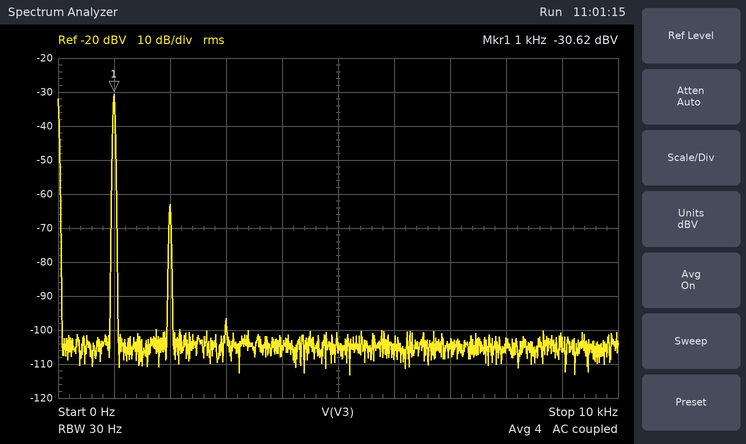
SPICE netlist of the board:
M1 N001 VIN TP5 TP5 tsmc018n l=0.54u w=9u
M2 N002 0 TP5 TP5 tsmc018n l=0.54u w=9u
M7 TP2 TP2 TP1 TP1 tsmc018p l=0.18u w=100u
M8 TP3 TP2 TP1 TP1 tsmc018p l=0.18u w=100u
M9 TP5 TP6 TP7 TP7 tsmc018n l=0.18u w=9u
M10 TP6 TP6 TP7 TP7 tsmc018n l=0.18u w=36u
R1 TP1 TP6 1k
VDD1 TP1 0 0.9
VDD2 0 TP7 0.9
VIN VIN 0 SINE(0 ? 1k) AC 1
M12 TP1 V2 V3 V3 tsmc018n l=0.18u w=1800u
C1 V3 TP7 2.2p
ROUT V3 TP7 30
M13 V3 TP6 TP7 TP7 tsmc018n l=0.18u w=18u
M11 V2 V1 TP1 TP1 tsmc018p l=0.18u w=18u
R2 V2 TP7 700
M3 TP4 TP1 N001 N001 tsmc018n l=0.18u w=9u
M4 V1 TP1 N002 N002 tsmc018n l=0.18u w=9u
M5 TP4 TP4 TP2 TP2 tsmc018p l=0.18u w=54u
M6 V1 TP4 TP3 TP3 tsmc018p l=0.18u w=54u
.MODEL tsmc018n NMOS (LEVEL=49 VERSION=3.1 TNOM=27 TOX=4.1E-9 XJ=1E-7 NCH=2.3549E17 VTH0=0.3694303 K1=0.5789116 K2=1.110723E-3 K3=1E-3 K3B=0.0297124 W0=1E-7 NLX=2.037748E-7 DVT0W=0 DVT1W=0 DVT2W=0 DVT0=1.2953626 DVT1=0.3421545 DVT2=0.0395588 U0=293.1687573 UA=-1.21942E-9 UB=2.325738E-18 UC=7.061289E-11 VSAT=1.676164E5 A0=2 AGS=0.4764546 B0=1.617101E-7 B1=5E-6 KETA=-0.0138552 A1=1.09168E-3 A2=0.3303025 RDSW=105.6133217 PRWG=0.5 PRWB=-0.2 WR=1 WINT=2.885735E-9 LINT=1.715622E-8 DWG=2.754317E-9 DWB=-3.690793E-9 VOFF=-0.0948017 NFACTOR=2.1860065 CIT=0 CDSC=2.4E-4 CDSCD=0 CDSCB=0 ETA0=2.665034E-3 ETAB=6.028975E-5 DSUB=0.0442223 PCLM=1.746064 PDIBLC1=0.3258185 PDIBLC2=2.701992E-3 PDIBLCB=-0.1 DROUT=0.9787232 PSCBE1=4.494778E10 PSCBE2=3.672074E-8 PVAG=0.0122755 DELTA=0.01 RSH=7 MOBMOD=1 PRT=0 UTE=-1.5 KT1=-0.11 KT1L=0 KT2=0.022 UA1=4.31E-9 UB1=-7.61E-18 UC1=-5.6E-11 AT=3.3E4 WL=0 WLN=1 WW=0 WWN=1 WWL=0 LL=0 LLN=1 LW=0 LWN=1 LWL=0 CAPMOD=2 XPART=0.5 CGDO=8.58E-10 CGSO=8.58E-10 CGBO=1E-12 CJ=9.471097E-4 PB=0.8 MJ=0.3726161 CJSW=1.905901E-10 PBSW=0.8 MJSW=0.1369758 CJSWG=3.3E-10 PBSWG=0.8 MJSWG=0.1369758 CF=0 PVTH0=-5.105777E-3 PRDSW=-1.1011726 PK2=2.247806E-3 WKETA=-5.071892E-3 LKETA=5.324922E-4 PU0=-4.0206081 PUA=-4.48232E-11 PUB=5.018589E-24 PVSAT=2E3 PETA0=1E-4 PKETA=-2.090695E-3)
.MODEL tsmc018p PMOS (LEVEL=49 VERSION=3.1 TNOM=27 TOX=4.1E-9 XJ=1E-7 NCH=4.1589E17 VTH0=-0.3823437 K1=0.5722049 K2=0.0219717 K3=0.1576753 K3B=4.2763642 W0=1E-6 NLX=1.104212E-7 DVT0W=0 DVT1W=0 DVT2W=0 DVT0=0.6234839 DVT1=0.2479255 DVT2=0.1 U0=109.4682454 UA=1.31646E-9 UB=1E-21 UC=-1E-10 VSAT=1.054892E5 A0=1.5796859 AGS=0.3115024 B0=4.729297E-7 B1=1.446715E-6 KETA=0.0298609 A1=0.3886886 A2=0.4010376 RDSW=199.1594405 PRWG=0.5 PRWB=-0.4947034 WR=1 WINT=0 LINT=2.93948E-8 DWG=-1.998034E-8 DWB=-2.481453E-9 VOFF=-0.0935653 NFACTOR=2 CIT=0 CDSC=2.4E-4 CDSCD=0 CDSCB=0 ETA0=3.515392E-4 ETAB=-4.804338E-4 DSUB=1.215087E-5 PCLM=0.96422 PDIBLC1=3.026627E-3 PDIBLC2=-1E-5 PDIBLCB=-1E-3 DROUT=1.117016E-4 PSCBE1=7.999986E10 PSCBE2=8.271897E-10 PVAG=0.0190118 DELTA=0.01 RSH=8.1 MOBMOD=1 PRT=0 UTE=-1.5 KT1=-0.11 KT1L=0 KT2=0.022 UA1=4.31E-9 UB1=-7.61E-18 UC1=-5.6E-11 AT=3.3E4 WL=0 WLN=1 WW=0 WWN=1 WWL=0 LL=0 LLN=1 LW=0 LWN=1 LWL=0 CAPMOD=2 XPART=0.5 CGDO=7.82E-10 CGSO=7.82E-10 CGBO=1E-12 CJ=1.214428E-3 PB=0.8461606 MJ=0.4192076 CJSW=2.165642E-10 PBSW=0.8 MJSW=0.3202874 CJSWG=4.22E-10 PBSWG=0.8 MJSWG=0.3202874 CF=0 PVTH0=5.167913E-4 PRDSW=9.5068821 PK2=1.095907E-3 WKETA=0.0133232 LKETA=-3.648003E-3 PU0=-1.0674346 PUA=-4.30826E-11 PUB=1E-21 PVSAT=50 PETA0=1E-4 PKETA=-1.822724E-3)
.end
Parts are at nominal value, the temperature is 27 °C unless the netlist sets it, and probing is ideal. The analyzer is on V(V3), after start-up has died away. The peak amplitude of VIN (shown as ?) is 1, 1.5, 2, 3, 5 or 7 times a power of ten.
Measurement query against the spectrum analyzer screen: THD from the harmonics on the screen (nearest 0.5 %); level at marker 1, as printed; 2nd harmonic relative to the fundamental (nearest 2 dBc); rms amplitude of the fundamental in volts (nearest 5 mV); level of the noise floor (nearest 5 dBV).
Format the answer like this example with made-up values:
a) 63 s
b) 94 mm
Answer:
a) 2.5 %
b) -30.62 dBV
c) -32 dBc
d) 30 mV
e) -105 dBV
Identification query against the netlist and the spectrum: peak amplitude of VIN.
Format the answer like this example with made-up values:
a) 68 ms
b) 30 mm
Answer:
a) 500 µV
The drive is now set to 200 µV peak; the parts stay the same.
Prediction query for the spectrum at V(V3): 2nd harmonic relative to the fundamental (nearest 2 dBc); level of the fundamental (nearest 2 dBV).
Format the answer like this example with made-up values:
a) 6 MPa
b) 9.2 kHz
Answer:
a) -40 dBc
b) -38 dBV
